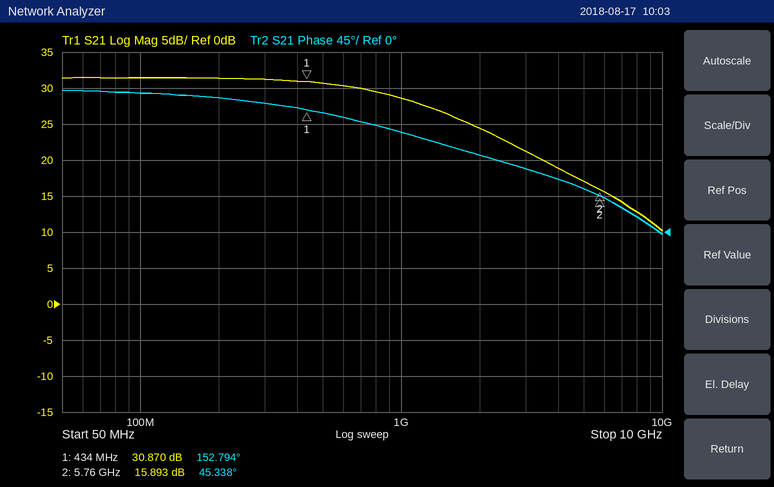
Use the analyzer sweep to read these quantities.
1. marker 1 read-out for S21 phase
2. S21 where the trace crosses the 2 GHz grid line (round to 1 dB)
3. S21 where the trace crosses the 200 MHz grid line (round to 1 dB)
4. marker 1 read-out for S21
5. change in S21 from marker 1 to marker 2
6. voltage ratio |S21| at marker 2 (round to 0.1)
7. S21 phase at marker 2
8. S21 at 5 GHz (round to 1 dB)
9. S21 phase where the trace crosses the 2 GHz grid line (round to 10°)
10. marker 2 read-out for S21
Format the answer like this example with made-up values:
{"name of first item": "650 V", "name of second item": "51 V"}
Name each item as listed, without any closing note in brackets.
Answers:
{"marker 1 read-out for S21 phase": "152.794°", "S21 where the trace crosses the 2 GHz grid line": "24 dB", "S21 where the trace crosses the 200 MHz grid line": "31 dB", "marker 1 read-out for S21": "30.870 dB", "change in S21 from marker 1 to marker 2": "-14.977 dB", "voltage ratio |S21| at marker 2": "6.2", "S21 phase at marker 2": "45.338°", "S21 at 5 GHz": "17 dB", "S21 phase where the trace crosses the 2 GHz grid line": "100°", "marker 2 read-out for S21": "15.893 dB"}
